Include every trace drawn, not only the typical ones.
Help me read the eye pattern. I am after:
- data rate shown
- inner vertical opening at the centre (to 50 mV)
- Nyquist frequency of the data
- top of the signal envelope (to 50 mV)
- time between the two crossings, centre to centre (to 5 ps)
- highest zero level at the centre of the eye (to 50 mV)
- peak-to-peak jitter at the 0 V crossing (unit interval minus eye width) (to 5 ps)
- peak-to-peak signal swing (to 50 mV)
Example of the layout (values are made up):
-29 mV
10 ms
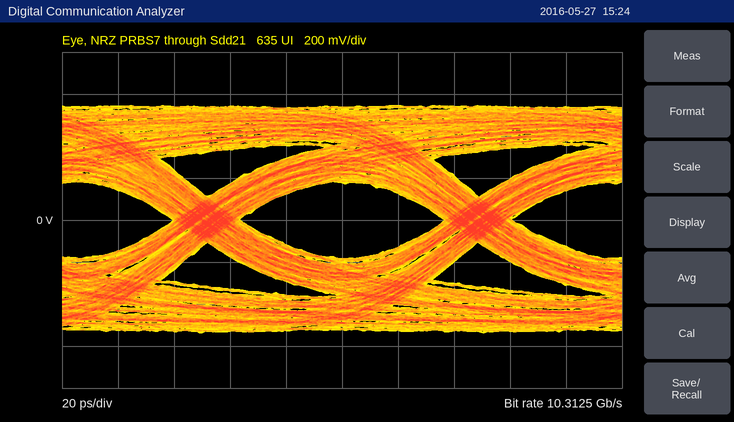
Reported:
10.3125 Gb/s
350 mV
5.15625 GHz
550 mV
95 ps
-200 mV
25 ps
1.10 V
